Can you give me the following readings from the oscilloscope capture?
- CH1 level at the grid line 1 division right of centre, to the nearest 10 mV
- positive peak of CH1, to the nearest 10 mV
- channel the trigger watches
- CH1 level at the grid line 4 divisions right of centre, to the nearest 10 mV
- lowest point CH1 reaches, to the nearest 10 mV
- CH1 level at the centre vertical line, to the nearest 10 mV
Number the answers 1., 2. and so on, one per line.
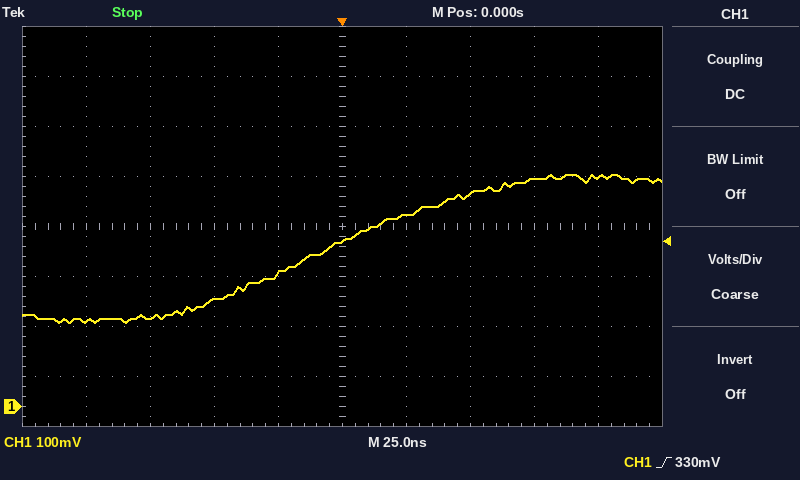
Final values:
1. 380 mV
2. 460 mV
3. CH1
4. 460 mV
5. 170 mV
6. 330 mV
